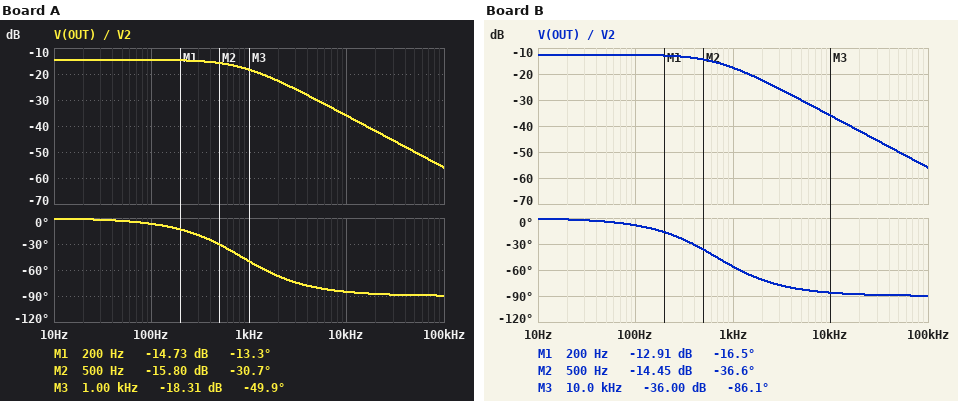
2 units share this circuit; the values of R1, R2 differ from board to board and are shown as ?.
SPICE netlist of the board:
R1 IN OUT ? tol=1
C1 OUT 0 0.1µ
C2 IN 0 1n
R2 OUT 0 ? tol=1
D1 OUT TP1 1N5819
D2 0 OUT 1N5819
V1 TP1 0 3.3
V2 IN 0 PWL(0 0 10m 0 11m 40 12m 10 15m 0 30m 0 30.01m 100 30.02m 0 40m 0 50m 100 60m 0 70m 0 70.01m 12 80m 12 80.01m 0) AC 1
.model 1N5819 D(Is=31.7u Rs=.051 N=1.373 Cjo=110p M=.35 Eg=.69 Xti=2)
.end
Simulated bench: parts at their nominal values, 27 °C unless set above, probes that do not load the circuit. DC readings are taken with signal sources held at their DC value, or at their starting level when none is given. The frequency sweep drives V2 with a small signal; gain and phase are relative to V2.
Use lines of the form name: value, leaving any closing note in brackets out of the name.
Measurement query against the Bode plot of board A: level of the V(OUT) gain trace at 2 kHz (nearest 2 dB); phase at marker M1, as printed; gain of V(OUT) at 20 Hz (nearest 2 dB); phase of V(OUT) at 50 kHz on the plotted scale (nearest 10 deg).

level of the V(OUT) gain trace at 2 kHz: -22 dB
phase at marker M1, as printed: -13.3 deg
gain of V(OUT) at 20 Hz: -14 dB
phase of V(OUT) at 50 kHz on the plotted scale: -90 deg
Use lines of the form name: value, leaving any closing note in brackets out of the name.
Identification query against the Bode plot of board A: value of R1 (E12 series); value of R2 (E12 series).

value of R1: 10 kΩ
value of R2: 6.8 kΩ
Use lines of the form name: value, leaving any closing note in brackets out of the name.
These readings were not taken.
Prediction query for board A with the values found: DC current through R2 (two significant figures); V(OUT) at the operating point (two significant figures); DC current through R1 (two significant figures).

DC current through R2: 6.0 µA
V(OUT) at the operating point: 41 mV
DC current through R1: 4.1 µA
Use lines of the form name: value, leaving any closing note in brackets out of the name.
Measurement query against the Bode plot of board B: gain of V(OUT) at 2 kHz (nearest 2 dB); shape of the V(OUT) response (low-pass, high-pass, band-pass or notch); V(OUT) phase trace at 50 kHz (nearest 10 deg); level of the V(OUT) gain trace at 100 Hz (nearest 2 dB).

gain of V(OUT) at 2 kHz: -22 dB
shape of the V(OUT) response: low-pass
V(OUT) phase trace at 50 kHz: -90 deg
level of the V(OUT) gain trace at 100 Hz: -12 dB
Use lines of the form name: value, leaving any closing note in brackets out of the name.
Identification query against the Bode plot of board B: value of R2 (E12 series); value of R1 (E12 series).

value of R2: 12 kΩ
value of R1: 10 kΩ
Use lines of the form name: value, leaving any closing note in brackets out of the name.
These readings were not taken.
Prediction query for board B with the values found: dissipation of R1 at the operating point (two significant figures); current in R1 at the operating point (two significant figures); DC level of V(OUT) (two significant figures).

dissipation of R1 at the operating point: 220 nW
current in R1 at the operating point: 4.7 µA
DC level of V(OUT): 47 mV
